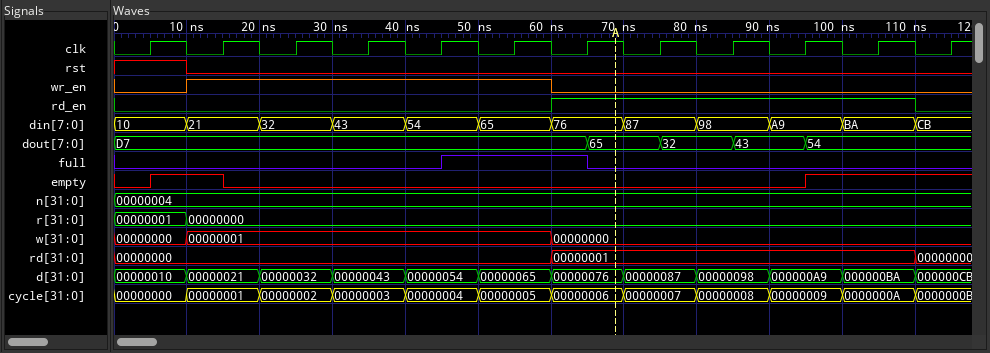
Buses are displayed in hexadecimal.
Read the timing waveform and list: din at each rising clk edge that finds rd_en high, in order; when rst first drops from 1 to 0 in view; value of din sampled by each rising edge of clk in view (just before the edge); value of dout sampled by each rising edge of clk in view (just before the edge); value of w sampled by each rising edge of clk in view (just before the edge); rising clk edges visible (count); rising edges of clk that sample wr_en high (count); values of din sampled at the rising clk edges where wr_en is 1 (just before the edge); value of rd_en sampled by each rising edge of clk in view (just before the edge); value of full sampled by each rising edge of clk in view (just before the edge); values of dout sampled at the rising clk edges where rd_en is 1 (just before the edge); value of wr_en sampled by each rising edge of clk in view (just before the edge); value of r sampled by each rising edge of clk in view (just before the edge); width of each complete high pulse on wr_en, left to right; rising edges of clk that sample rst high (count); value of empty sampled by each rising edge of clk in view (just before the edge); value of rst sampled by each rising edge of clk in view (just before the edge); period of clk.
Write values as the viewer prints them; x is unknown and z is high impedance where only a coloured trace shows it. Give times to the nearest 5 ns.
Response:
76, 87, 98, A9, BA
10 ns
10, 21, 32, 43, 54, 65, 76, 87, 98, A9, BA, CB
D7, D7, D7, D7, D7, D7, D7, 65, 32, 43, 54, 54
00000000, 00000001, 00000001, 00000001, 00000001, 00000001, 00000000, 00000000, 00000000, 00000000, 00000000, 00000000
12
5
21, 32, 43, 54, 65
0 0 0 0 0 0 1 1 1 1 1 0
0 0 0 0 0 1 1 0 0 0 0 0
D7, 65, 32, 43, 54
0 1 1 1 1 1 0 0 0 0 0 0
00000001, 00000000, 00000000, 00000000, 00000000, 00000000, 00000000, 00000000, 00000000, 00000000, 00000000, 00000000
50 ns
1
0 1 0 0 0 0 0 0 0 0 1 1
1 0 0 0 0 0 0 0 0 0 0 0
10 ns
